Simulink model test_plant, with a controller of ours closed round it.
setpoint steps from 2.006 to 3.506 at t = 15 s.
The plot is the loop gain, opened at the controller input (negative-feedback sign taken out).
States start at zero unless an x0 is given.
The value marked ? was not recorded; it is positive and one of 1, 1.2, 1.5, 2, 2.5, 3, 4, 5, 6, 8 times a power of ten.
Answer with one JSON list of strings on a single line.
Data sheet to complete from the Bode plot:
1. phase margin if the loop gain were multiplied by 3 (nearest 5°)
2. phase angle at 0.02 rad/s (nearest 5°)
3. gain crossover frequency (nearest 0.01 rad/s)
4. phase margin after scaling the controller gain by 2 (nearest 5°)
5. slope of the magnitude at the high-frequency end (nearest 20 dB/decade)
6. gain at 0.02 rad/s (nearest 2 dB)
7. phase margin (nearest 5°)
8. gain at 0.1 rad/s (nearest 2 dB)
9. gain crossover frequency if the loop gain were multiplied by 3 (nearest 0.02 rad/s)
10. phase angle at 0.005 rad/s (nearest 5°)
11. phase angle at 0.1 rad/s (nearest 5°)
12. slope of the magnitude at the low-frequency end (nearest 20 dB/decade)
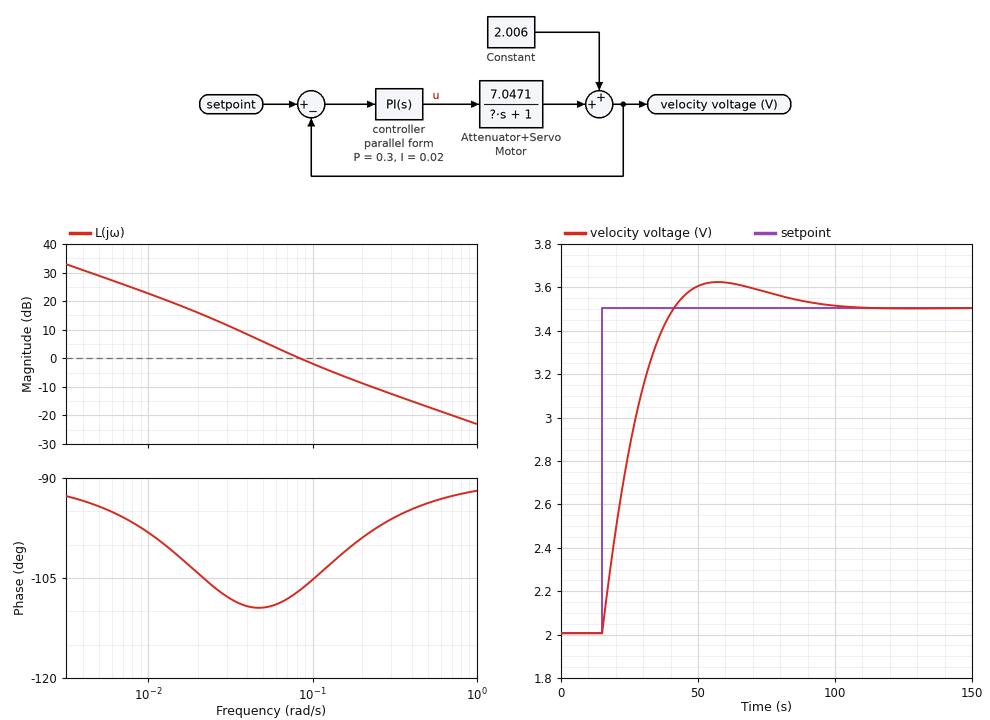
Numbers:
["80°", "-105°", "0.08 rad/s", "80°", "-20 dB/decade", "16 dB", "75°", "-2 dB", "0.22 rad/s", "-95°", "-105°", "-20 dB/decade"]
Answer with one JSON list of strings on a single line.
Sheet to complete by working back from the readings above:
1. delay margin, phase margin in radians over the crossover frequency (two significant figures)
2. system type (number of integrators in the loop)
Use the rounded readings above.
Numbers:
["16 s", "1"]
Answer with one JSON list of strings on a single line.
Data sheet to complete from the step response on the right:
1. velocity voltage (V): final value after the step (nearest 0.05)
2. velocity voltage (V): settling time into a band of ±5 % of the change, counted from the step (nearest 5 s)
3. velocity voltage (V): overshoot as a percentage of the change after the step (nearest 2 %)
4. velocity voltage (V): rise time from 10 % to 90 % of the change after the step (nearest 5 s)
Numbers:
["3.50", "60 s", "8 %", "20 s"]
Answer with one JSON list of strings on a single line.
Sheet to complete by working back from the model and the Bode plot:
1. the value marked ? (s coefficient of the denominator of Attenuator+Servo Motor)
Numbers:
["30"]
